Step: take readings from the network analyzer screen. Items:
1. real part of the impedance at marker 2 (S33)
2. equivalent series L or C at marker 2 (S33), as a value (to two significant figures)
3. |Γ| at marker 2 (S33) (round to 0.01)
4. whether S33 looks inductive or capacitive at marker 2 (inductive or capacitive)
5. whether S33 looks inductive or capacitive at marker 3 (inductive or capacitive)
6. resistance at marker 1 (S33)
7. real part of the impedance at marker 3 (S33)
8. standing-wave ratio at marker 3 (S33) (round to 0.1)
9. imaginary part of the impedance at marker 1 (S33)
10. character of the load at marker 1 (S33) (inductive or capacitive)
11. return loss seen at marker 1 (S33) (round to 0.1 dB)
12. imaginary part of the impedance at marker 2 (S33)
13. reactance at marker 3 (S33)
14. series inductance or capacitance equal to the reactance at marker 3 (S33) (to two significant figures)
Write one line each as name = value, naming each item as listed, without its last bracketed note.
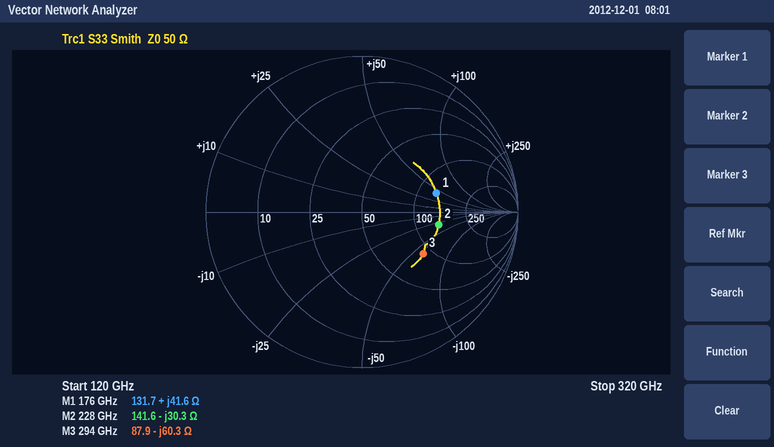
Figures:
real part of the impedance at marker 2 = 141.6 Ω
equivalent series L or C at marker 2 (S33), as a value = 23 fF
|Γ| at marker 2 (S33) = 0.50
whether S33 looks inductive or capacitive at marker 2 = capacitive
whether S33 looks inductive or capacitive at marker 3 = capacitive
resistance at marker 1 = 131.7 Ω
real part of the impedance at marker 3 = 87.9 Ω
standing-wave ratio at marker 3 (S33) = 2.8
imaginary part of the impedance at marker 1 = +41.6 Ω
character of the load at marker 1 (S33) = inductive
return loss seen at marker 1 (S33) = 6.2 dB
imaginary part of the impedance at marker 2 = -30.3 Ω
reactance at marker 3 = -60.3 Ω
series inductance or capacitance equal to the reactance at marker 3 (S33) = 9.0 fF
